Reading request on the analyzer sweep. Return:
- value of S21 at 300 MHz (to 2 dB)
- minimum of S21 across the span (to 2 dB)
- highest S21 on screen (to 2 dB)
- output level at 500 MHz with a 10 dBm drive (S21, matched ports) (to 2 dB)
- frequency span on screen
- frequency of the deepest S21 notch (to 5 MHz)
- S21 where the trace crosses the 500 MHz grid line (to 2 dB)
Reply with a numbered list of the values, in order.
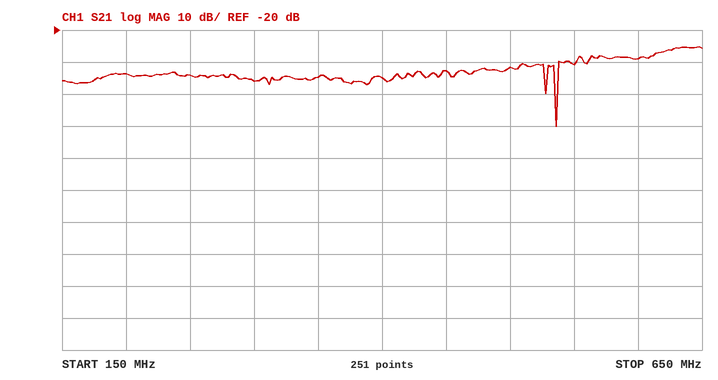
1. -36 dB
2. -50 dB
3. -26 dB
4. -22 dBm
5. 500 MHz
6. 535 MHz
7. -32 dB
